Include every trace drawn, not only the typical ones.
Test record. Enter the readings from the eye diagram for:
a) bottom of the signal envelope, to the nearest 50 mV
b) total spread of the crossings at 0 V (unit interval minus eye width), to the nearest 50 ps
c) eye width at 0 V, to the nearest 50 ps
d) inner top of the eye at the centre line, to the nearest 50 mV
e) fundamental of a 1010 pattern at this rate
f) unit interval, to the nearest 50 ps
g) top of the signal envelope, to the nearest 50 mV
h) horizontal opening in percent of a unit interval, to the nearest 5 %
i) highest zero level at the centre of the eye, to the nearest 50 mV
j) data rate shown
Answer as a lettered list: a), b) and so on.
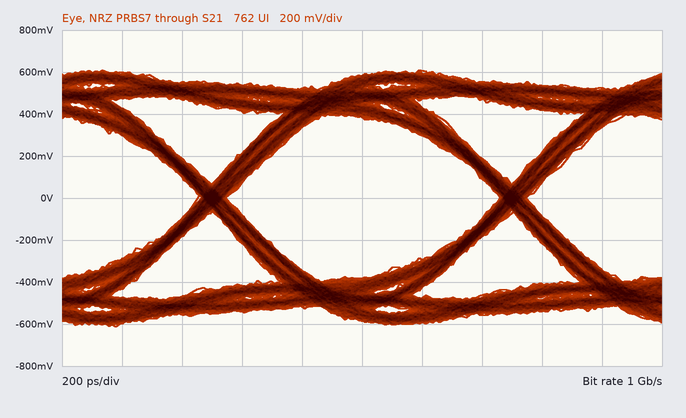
a) -600 mV
b) 100 ps
c) 900 ps
d) 400 mV
e) 500 MHz
f) 1.00 ns
g) 600 mV
h) 90 %
i) -400 mV
j) 1 Gb/s
